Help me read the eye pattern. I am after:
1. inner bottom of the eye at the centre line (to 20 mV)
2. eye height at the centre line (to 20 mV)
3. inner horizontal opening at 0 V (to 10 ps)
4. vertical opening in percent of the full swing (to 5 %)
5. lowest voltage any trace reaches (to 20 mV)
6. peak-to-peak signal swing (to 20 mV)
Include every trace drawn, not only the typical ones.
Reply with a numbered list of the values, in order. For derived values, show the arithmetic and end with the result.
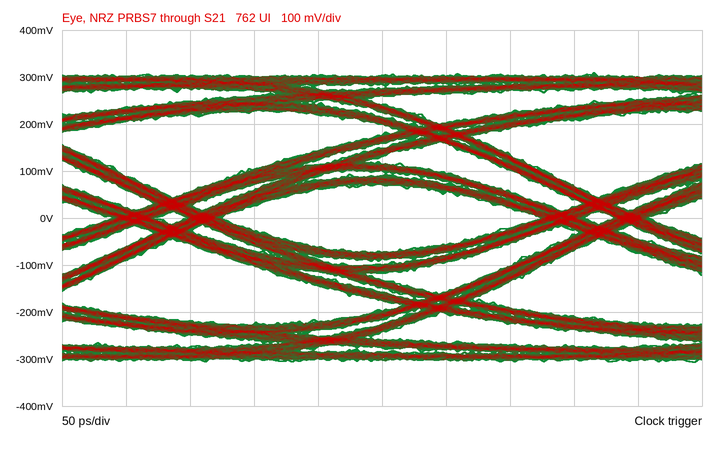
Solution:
1. -80 mV
2. 140 mV
3. 250 ps
4. 140 mV / 620 mV ≈ 22.6 %, so 25 % to the nearest 5 %
5. -300 mV
6. 620 mV
